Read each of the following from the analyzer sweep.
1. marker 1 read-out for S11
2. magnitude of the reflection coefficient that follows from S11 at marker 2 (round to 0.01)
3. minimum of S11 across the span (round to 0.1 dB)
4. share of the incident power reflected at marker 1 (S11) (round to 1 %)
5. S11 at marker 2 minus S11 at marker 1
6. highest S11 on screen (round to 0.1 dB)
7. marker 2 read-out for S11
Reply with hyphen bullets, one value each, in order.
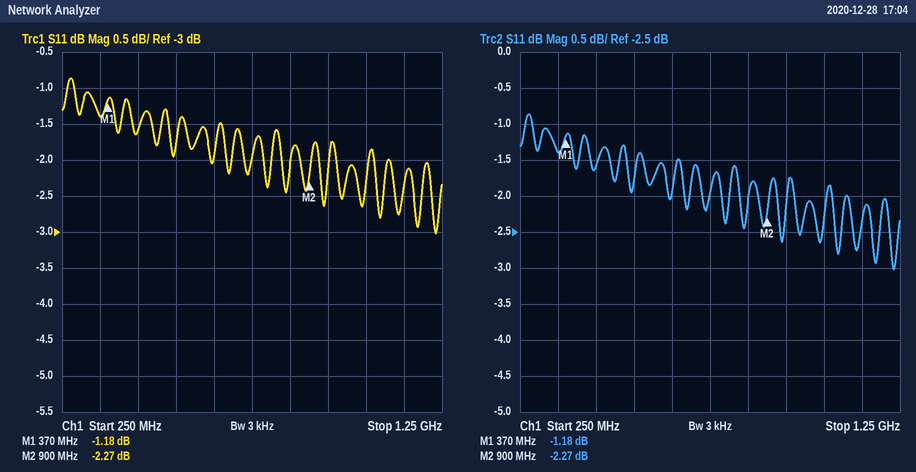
- -1.18 dB
- 0.77
- -3.0 dB
- 76 %
- -1.09 dB
- -0.9 dB
- -2.27 dB
